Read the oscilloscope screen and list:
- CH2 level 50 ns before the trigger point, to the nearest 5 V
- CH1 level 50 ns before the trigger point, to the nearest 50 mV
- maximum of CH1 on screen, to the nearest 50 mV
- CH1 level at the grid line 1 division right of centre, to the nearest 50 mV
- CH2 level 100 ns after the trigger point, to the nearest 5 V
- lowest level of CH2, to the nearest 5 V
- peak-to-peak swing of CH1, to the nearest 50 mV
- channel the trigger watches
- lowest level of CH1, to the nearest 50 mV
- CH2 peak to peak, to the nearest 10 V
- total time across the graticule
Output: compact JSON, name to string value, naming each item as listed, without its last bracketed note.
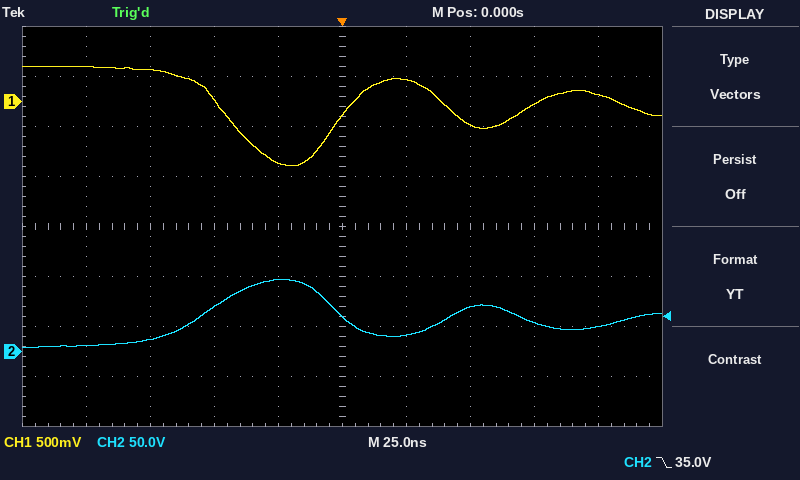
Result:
{"CH2 level 50 ns before the trigger point, to the nearest 5 V": "45 V", "CH1 level 50 ns before the trigger point, to the nearest 50 mV": "0 mV", "maximum of CH1 on screen, to the nearest 50 mV": "350 mV", "CH1 level at the grid line 1 division right of centre, to the nearest 50 mV": "200 mV", "CH2 level 100 ns after the trigger point, to the nearest 5 V": "25 V", "lowest level of CH2, to the nearest 5 V": "5 V", "peak-to-peak swing of CH1, to the nearest 50 mV": "1.00 V", "channel the trigger watches": "CH2", "lowest level of CH1, to the nearest 50 mV": "-650 mV", "CH2 peak to peak, to the nearest 10 V": "70 V", "total time across the graticule": "250 ns"}
